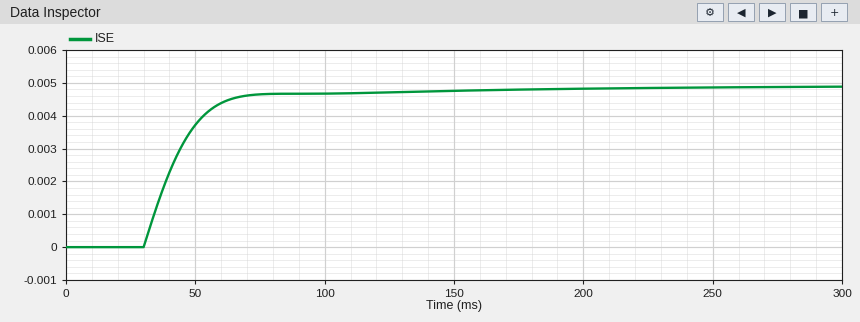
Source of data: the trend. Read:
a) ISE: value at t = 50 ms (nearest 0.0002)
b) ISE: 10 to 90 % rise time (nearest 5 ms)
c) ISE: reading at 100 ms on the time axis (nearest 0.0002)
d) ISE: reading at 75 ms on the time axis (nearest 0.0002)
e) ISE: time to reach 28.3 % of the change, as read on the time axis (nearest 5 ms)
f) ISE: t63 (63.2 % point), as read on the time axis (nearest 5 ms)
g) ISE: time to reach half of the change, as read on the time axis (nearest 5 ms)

0.0038
30 ms
0.0046
0.0046
35 ms
45 ms
40 ms
